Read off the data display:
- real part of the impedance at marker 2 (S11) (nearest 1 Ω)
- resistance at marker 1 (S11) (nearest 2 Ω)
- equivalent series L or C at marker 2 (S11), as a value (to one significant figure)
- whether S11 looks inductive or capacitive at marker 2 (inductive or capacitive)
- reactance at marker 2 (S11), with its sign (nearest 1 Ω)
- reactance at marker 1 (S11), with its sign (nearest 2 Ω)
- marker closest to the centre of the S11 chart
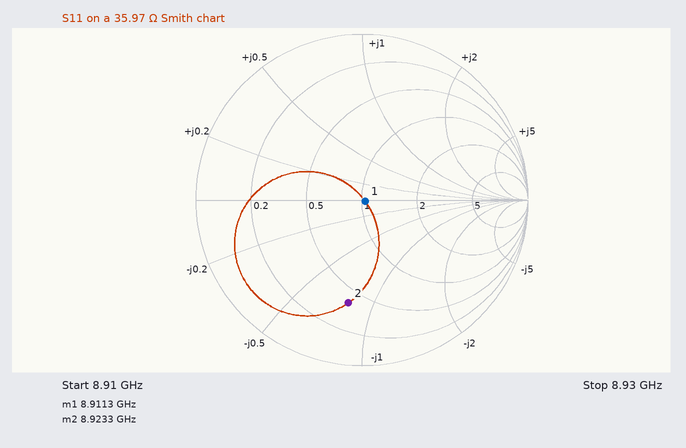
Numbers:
14 Ω
38 Ω
600 fF
capacitive
-29 Ω
0 Ω
marker 1
